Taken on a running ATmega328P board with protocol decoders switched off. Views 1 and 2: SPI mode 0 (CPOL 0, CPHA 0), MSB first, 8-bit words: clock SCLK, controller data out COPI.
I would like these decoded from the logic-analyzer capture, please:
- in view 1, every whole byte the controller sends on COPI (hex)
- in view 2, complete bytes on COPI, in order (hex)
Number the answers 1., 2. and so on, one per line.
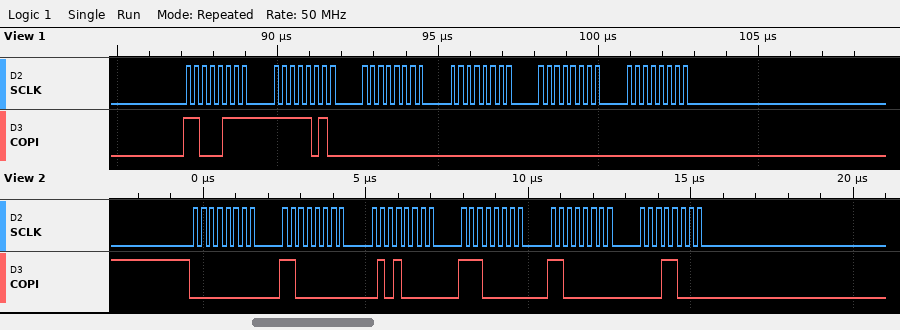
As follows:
1. 0xC7 0xFA 0x00 0x00 0x00 0x00
2. 00 C0 50 E0 C0 18
